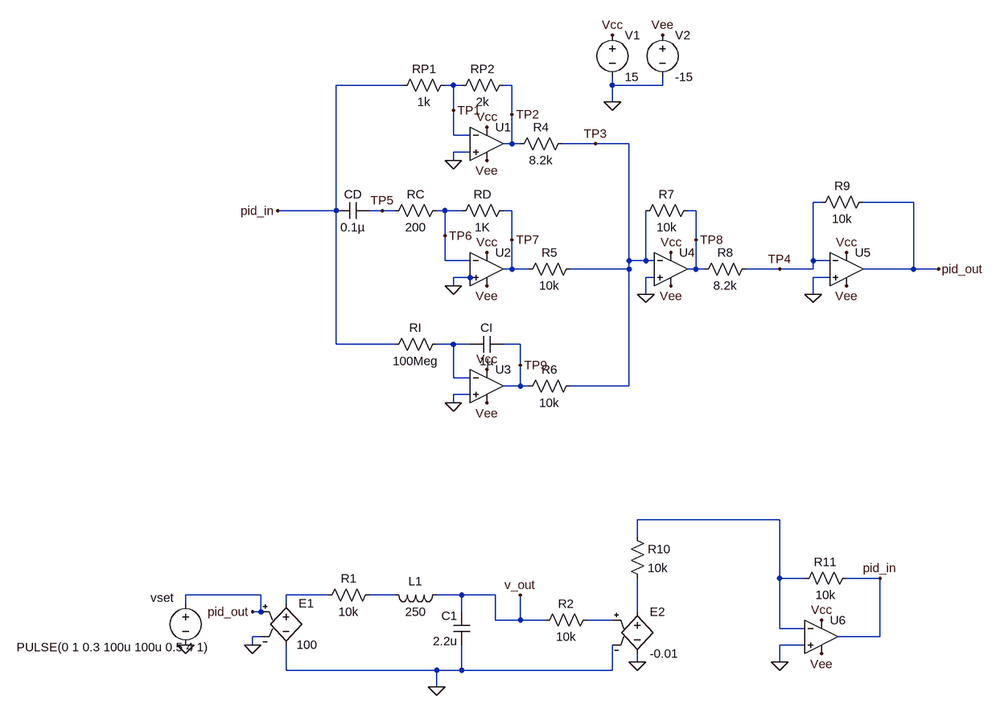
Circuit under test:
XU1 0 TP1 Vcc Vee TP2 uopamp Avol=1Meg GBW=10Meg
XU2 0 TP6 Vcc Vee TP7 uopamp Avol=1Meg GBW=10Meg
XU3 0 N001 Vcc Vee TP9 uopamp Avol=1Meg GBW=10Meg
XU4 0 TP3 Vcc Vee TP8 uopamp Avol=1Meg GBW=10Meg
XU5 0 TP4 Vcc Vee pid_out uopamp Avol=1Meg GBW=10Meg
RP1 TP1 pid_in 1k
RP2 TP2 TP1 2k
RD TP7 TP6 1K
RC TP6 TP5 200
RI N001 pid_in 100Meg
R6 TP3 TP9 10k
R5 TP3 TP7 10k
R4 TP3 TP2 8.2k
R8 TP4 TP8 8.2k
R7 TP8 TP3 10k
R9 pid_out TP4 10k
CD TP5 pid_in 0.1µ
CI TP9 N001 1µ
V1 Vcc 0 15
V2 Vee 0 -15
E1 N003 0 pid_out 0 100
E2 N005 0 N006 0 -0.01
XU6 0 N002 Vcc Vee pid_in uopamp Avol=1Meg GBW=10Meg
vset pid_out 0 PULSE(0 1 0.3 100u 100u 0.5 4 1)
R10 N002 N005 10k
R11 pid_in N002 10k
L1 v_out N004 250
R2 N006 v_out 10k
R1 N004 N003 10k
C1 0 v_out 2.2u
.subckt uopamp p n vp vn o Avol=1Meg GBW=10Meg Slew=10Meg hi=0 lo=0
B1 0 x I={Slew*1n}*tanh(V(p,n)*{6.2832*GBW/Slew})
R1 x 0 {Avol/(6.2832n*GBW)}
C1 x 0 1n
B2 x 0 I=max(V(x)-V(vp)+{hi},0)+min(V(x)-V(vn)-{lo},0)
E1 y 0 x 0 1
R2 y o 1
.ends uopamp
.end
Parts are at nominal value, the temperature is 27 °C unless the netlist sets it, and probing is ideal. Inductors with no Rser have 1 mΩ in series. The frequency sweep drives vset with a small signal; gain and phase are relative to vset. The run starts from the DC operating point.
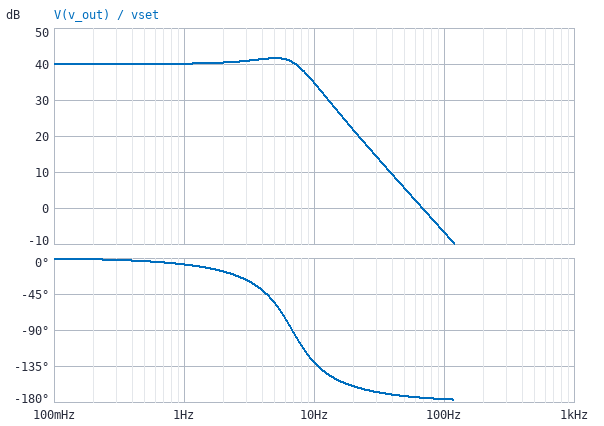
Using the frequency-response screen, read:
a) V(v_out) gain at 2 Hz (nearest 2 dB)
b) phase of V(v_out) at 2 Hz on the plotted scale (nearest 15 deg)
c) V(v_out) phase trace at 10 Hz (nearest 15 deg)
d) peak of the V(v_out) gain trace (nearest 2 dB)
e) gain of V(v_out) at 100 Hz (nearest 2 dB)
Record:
40 dB
-15 deg
-135 deg
42 dB
-6 dB
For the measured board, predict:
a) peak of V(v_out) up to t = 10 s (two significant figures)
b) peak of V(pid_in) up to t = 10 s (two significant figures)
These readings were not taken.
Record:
120 V
1.2 V
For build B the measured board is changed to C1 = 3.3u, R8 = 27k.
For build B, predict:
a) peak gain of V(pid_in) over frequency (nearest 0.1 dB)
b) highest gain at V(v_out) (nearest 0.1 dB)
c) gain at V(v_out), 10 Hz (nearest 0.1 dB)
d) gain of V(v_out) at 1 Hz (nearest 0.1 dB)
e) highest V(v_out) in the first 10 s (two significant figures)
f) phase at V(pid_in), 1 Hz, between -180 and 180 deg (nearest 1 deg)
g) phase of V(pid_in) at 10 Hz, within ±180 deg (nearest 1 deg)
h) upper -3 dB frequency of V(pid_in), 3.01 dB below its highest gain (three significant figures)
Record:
0.5 dB
40.5 dB
30.3 dB
40.1 dB
110 V
-12 deg
-137 deg
6.27 Hz
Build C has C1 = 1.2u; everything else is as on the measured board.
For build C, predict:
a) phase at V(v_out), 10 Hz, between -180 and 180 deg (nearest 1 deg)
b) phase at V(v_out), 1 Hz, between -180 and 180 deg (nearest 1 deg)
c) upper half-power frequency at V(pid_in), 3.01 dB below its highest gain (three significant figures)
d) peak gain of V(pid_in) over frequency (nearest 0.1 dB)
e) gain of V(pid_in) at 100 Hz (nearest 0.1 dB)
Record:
-104 deg
-4 deg
10.9 Hz
3.7 dB
-41.4 dB
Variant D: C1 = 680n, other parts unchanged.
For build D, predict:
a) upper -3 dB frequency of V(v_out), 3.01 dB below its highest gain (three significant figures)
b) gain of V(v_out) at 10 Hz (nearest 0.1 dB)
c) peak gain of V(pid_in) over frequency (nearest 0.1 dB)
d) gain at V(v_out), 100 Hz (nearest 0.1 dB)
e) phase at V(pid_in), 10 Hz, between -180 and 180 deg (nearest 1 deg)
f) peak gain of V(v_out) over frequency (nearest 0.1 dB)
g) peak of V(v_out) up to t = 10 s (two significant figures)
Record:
14.3 Hz
45.4 dB
6.0 dB
3.6 dB
-52 deg
46.0 dB
140 V
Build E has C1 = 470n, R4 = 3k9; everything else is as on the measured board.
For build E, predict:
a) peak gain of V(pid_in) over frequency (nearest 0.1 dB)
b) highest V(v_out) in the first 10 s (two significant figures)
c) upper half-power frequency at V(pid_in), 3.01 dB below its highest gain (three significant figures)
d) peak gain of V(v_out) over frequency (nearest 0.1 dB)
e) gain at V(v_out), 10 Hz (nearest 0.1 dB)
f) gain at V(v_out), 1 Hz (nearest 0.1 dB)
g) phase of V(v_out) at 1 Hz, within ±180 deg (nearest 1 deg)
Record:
7.5 dB
150 V
16.9 Hz
47.5 dB
44.3 dB
40.0 dB
-2 deg
